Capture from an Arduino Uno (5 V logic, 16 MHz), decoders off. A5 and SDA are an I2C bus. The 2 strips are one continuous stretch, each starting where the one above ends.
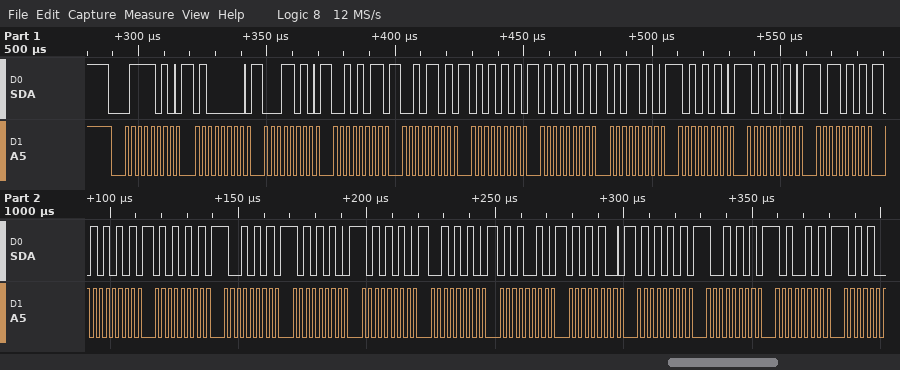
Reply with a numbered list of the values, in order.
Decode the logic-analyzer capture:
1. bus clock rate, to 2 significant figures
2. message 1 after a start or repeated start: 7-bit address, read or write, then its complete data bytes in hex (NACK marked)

1. 400 kHz
2. 0x3D write: 40 1A 2B 2D 55 55 5A AA AA B5 55 55 95 AA AA 2A 52 54 55 95 A5
